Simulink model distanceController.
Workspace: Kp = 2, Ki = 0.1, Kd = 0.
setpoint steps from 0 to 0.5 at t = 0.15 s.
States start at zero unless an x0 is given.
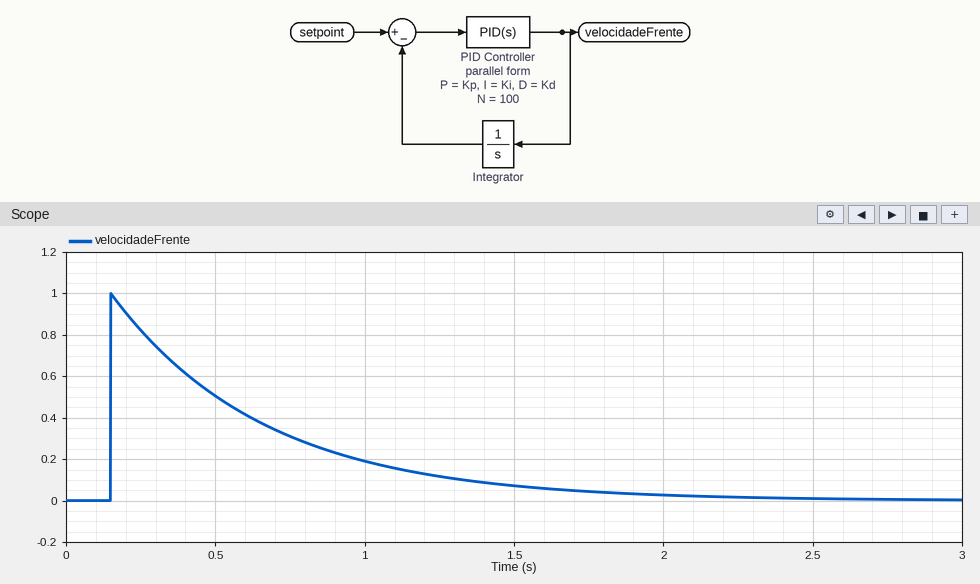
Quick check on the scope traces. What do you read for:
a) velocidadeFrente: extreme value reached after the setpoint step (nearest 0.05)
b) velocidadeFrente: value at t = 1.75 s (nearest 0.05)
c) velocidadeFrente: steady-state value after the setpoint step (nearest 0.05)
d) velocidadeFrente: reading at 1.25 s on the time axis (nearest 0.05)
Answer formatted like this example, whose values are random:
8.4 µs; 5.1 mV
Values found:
1.00; 0.05; 0.00; 0.10
